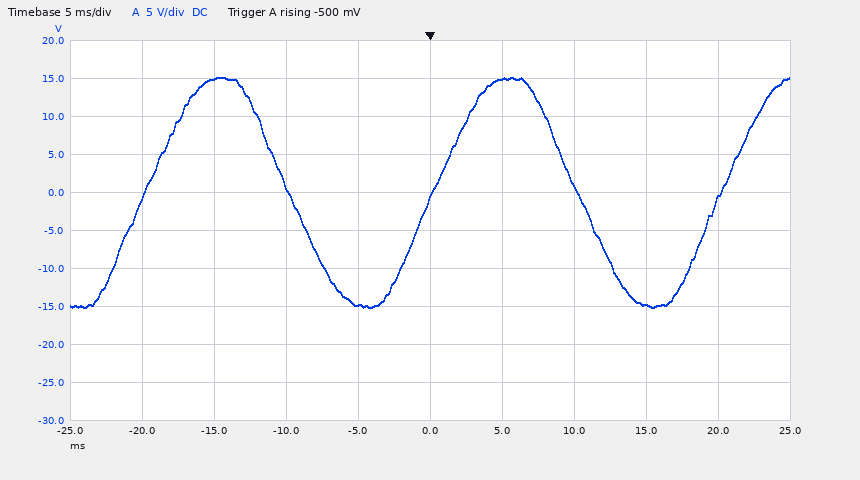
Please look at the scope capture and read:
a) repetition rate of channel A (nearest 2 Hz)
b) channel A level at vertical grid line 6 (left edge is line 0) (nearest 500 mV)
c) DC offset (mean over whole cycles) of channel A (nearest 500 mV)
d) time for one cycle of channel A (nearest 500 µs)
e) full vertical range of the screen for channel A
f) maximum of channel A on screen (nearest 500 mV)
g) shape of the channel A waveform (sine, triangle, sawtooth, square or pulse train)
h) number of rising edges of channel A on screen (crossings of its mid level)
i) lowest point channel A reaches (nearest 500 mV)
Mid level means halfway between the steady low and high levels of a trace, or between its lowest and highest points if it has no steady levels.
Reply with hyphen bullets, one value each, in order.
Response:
- 50 Hz
- 15.0 V
- 0.0 V
- 20.0 ms
- 50 V
- 15.0 V
- sine
- 3
- -15.0 V
